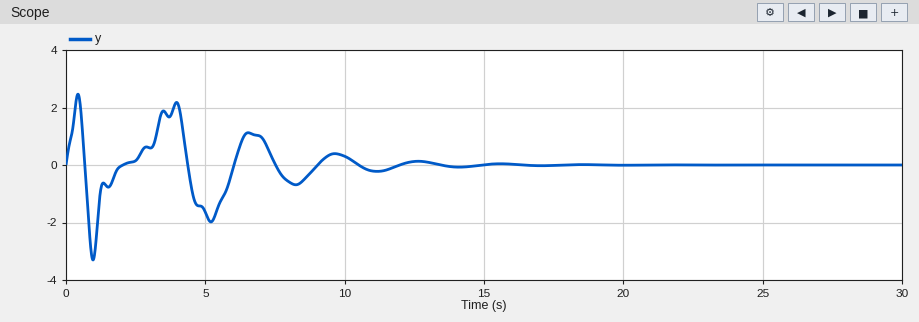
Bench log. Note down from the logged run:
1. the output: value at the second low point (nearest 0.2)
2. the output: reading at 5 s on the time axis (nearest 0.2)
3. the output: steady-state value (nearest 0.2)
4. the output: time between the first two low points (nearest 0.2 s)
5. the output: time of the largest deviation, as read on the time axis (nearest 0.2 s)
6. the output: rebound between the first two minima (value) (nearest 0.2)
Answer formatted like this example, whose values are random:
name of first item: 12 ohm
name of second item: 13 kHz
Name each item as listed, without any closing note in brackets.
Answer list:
the output: value at the second low point: -2.0
the output: reading at 5 s on the time axis: -1.6
the output: steady-state value: 0.0
the output: time between the first two low points: 4.2 s
the output: time of the largest deviation, as read on the time axis: 1.0 s
the output: rebound between the first two minima (value): 2.2
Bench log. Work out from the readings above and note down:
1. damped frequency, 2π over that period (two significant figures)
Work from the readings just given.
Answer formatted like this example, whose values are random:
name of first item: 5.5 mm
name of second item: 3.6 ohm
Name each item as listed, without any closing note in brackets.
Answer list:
damped frequency, 2π over that period: 1.5 rad/s
